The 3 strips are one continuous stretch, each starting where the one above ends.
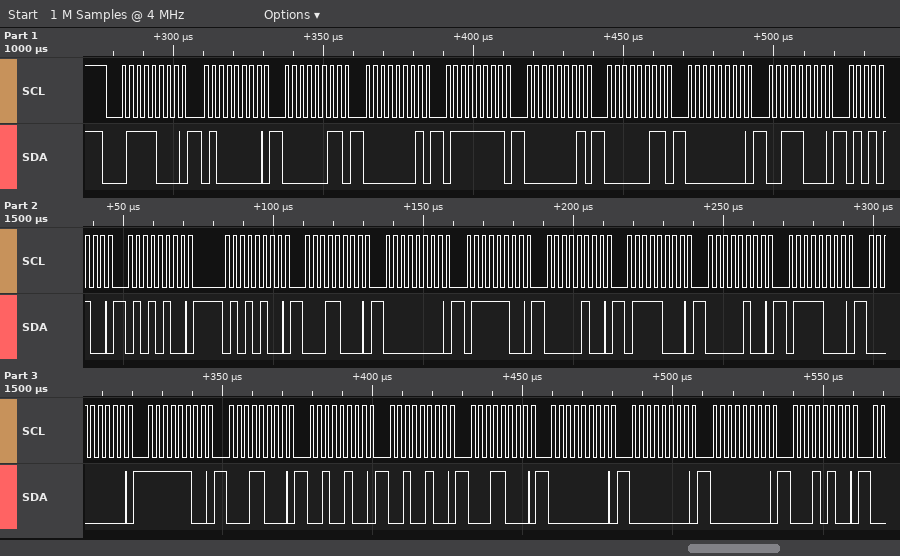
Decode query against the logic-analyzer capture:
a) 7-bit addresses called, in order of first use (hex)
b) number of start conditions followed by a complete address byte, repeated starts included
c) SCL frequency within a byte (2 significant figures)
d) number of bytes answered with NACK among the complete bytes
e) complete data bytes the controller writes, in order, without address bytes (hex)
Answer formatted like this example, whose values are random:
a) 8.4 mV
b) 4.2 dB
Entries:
a) 0x3C
b) 1
c) 400 kHz
d) 0
e) 40 03 01 7F 01 03 00 38 54 54 54 18 00 7C 04 78 04 78 00 FC 18 24 24 18 00 00 00 14
